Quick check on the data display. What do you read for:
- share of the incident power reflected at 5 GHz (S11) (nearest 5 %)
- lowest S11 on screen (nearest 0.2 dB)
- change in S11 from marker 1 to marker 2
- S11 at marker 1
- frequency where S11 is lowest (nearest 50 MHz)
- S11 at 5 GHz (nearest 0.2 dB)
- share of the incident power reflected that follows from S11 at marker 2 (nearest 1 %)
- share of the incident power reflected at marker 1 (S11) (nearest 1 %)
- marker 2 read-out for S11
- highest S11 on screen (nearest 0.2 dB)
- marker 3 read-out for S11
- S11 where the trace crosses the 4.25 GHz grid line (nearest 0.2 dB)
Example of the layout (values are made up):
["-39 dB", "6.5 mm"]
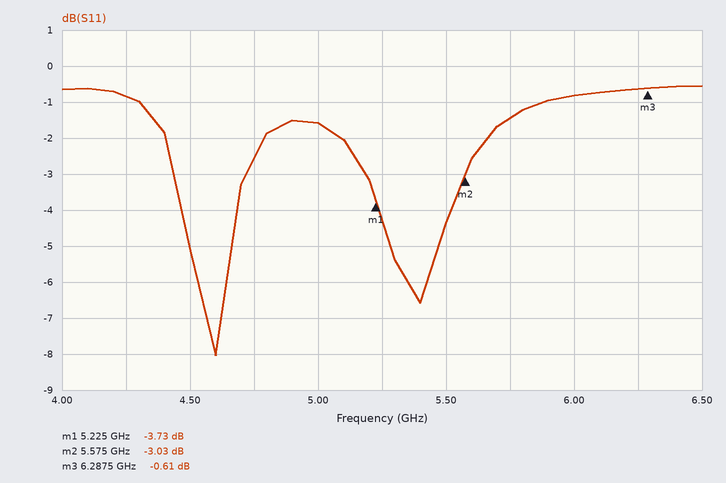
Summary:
["70 %", "-8.0 dB", "0.70 dB", "-3.73 dB", "4.60 GHz", "-1.6 dB", "50 %", "42 %", "-3.03 dB", "-0.6 dB", "-0.61 dB", "-0.8 dB"]
